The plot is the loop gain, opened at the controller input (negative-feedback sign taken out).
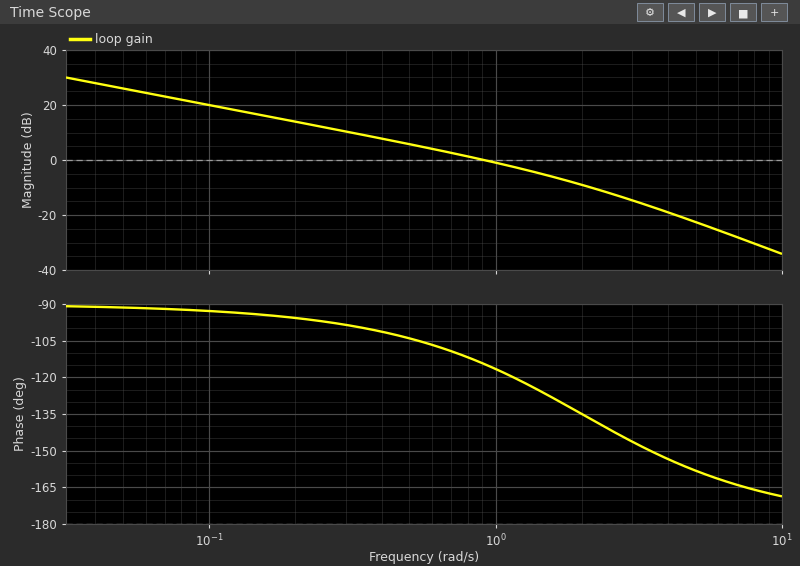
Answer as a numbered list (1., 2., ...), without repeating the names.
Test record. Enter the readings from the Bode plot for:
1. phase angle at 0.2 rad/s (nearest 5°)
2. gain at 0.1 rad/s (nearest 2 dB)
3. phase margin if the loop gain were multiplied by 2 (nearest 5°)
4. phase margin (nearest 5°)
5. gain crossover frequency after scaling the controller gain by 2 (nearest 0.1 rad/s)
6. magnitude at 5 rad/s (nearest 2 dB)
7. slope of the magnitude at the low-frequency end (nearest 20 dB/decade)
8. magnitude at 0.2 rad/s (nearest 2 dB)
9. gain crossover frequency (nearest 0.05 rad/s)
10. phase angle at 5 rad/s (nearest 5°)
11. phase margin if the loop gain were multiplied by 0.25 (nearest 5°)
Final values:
1. -95°
2. 20 dB
3. 50°
4. 65°
5. 1.6 rad/s
6. -22 dB
7. -20 dB/decade
8. 14 dB
9. 0.90 rad/s
10. -160°
11. 85°
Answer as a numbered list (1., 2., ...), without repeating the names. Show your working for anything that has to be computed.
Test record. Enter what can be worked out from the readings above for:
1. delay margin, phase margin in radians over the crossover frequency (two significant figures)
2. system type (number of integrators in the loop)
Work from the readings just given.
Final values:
1. 65 × π / 180 / 0.9 = 1.3 s
2. 1
